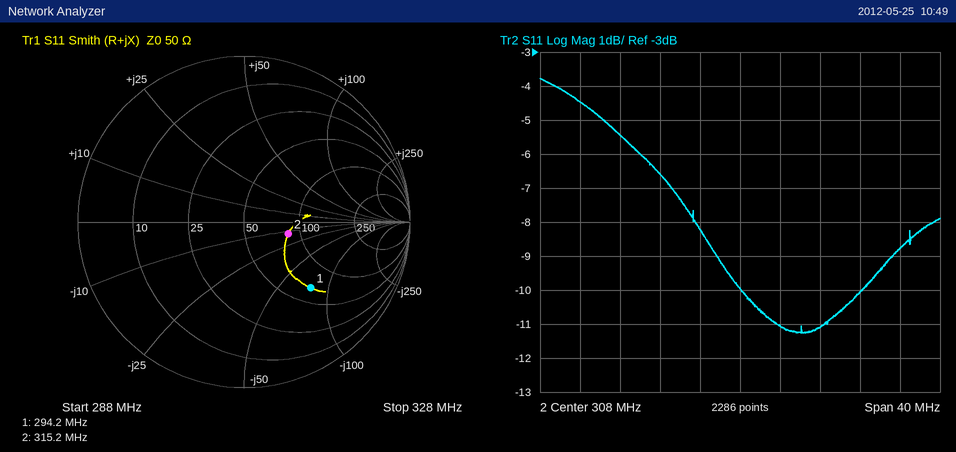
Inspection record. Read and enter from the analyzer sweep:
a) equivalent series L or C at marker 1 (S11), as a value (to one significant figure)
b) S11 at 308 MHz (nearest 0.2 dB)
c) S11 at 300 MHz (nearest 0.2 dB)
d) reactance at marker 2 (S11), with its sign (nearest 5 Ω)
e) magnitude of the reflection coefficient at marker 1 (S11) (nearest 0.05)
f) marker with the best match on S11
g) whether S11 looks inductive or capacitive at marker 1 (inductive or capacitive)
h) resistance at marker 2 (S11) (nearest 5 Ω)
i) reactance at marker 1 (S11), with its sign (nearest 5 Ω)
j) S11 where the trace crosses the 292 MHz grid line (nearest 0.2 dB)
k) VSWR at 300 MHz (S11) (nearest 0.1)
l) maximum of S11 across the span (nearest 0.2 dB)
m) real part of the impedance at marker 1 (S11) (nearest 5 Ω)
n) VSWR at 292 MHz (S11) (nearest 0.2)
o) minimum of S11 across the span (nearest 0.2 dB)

7 pF
-10.0 dB
-6.6 dB
-15 Ω
0.55
marker 2
capacitive
85 Ω
-75 Ω
-4.4 dB
2.8
-3.8 dB
65 Ω
4.0
-11.2 dB
